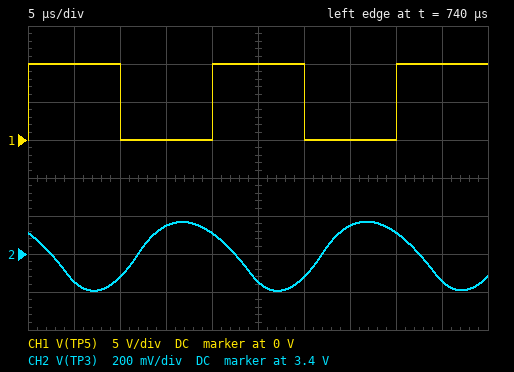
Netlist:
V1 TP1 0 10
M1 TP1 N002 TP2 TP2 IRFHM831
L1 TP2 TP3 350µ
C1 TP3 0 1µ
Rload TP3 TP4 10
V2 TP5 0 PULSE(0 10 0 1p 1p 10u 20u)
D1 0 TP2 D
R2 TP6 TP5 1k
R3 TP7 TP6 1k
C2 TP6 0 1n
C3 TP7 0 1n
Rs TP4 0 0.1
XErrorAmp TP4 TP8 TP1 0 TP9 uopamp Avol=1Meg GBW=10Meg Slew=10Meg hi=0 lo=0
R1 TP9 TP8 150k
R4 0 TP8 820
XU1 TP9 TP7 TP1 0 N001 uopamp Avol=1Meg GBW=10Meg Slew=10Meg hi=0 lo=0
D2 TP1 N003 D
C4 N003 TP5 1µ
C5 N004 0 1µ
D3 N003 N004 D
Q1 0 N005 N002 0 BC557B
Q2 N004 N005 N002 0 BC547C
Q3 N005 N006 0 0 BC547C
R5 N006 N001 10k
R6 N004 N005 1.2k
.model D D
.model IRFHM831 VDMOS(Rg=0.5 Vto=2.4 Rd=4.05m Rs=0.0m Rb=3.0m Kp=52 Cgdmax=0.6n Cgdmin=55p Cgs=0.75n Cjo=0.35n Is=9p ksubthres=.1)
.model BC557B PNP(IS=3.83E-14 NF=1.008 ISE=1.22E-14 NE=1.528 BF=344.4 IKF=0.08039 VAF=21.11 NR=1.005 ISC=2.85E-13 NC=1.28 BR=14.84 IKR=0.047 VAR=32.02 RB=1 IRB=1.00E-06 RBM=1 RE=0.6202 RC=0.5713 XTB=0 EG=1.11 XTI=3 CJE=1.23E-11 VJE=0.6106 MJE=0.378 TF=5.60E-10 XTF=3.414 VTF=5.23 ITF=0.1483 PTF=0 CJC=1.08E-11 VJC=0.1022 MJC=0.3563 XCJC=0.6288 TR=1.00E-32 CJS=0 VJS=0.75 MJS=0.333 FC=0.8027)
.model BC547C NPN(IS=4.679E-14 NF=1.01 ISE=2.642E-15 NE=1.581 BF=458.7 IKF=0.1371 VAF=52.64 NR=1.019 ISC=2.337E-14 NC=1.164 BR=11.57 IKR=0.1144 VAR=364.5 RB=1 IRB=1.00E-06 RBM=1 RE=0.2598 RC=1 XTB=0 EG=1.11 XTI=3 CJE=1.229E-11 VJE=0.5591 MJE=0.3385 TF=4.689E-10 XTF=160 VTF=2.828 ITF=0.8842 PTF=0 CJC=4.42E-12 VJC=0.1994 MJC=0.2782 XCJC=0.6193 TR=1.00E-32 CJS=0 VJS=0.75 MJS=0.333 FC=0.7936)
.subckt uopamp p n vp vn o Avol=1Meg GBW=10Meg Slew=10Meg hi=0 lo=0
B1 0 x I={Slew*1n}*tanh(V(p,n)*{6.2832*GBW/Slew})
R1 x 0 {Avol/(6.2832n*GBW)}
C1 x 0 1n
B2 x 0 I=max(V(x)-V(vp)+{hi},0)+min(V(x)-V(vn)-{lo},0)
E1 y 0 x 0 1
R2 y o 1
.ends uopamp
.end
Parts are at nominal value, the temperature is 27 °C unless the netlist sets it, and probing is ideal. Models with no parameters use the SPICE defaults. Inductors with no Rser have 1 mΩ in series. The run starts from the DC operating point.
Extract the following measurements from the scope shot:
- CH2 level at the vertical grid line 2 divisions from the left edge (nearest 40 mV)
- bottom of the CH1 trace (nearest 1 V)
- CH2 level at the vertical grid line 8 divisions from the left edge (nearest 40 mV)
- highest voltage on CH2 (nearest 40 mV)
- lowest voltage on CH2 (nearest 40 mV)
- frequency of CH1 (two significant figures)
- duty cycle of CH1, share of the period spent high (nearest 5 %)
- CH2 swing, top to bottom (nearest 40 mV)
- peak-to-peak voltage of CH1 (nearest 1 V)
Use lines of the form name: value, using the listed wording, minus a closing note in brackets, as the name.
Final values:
CH2 level at the vertical grid line 2 divisions from the left edge: 3.28 V
bottom of the CH1 trace: 0 V
CH2 level at the vertical grid line 8 divisions from the left edge: 3.52 V
highest voltage on CH2: 3.56 V
lowest voltage on CH2: 3.20 V
frequency of CH1: 50 kHz
duty cycle of CH1, share of the period spent high: 50 %
CH2 swing, top to bottom: 360 mV
peak-to-peak voltage of CH1: 10 V
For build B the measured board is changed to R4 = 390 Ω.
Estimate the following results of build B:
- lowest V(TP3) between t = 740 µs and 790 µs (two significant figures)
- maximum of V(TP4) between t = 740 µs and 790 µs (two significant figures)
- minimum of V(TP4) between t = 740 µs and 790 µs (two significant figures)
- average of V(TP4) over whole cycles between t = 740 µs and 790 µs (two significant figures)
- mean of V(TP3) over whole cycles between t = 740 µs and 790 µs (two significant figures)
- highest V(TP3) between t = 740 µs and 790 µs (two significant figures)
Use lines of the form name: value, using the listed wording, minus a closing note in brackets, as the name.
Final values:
lowest V(TP3) between t = 740 µs and 790 µs: 1.9 V
maximum of V(TP4) between t = 740 µs and 790 µs: 22 mV
minimum of V(TP4) between t = 740 µs and 790 µs: 19 mV
average of V(TP4) over whole cycles between t = 740 µs and 790 µs: 21 mV
mean of V(TP3) over whole cycles between t = 740 µs and 790 µs: 2.1 V
highest V(TP3) between t = 740 µs and 790 µs: 2.2 V
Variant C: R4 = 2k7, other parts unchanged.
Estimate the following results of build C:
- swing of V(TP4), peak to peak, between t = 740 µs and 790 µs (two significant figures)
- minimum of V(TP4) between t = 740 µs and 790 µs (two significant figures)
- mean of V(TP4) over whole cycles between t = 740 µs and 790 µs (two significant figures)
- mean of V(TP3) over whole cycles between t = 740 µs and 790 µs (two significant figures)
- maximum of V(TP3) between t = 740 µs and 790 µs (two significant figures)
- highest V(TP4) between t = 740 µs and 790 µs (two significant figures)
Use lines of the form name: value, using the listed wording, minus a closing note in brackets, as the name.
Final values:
swing of V(TP4), peak to peak, between t = 740 µs and 790 µs: 3.7 mV
minimum of V(TP4) between t = 740 µs and 790 µs: 51 mV
mean of V(TP4) over whole cycles between t = 740 µs and 790 µs: 53 mV
mean of V(TP3) over whole cycles between t = 740 µs and 790 µs: 5.3 V
maximum of V(TP3) between t = 740 µs and 790 µs: 5.5 V
highest V(TP4) between t = 740 µs and 790 µs: 55 mV
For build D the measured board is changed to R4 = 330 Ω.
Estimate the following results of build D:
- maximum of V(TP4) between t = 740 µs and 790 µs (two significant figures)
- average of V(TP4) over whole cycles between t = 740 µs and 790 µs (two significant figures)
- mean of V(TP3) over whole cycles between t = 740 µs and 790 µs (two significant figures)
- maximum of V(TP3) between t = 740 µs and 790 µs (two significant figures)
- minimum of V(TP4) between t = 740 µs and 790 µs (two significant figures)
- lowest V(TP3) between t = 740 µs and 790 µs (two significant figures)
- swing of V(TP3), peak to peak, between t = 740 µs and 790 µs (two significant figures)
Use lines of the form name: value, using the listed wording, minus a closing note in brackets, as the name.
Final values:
maximum of V(TP4) between t = 740 µs and 790 µs: 19 mV
average of V(TP4) over whole cycles between t = 740 µs and 790 µs: 18 mV
mean of V(TP3) over whole cycles between t = 740 µs and 790 µs: 1.8 V
maximum of V(TP3) between t = 740 µs and 790 µs: 1.9 V
minimum of V(TP4) between t = 740 µs and 790 µs: 16 mV
lowest V(TP3) between t = 740 µs and 790 µs: 1.7 V
swing of V(TP3), peak to peak, between t = 740 µs and 790 µs: 280 mV
